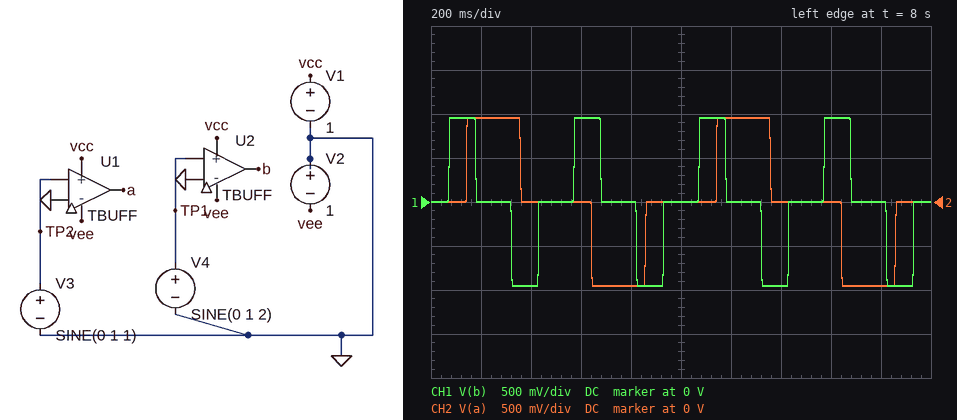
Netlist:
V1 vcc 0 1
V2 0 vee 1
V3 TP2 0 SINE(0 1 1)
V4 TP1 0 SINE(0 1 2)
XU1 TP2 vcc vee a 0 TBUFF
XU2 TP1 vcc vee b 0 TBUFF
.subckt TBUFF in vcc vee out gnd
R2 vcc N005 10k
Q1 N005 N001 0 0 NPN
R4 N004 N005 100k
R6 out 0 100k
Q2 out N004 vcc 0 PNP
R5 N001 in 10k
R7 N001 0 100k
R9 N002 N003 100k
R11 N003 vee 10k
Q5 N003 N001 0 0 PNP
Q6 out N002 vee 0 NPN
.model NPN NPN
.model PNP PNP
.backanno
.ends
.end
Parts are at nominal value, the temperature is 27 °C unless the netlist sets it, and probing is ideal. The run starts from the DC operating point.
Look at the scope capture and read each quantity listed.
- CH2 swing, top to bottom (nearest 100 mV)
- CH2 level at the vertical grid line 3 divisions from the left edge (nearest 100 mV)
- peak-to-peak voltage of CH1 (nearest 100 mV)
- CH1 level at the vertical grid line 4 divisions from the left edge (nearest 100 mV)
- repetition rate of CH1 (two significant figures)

1.9 V
0 V
1.9 V
0 V
2.0 Hz
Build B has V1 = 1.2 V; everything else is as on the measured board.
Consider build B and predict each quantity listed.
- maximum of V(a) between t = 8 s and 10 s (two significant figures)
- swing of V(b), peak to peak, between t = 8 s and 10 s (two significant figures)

1.2 V
2.1 V
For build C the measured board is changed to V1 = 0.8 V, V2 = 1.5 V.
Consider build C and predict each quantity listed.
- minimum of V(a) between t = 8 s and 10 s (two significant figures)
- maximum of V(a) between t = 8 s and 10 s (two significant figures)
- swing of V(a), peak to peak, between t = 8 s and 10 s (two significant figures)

-1.5 V
740 mV
2.2 V
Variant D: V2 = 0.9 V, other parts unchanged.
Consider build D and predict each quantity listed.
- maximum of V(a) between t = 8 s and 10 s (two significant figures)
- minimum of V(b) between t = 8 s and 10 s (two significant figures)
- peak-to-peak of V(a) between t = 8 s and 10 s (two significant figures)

960 mV
-850 mV
1.8 V
